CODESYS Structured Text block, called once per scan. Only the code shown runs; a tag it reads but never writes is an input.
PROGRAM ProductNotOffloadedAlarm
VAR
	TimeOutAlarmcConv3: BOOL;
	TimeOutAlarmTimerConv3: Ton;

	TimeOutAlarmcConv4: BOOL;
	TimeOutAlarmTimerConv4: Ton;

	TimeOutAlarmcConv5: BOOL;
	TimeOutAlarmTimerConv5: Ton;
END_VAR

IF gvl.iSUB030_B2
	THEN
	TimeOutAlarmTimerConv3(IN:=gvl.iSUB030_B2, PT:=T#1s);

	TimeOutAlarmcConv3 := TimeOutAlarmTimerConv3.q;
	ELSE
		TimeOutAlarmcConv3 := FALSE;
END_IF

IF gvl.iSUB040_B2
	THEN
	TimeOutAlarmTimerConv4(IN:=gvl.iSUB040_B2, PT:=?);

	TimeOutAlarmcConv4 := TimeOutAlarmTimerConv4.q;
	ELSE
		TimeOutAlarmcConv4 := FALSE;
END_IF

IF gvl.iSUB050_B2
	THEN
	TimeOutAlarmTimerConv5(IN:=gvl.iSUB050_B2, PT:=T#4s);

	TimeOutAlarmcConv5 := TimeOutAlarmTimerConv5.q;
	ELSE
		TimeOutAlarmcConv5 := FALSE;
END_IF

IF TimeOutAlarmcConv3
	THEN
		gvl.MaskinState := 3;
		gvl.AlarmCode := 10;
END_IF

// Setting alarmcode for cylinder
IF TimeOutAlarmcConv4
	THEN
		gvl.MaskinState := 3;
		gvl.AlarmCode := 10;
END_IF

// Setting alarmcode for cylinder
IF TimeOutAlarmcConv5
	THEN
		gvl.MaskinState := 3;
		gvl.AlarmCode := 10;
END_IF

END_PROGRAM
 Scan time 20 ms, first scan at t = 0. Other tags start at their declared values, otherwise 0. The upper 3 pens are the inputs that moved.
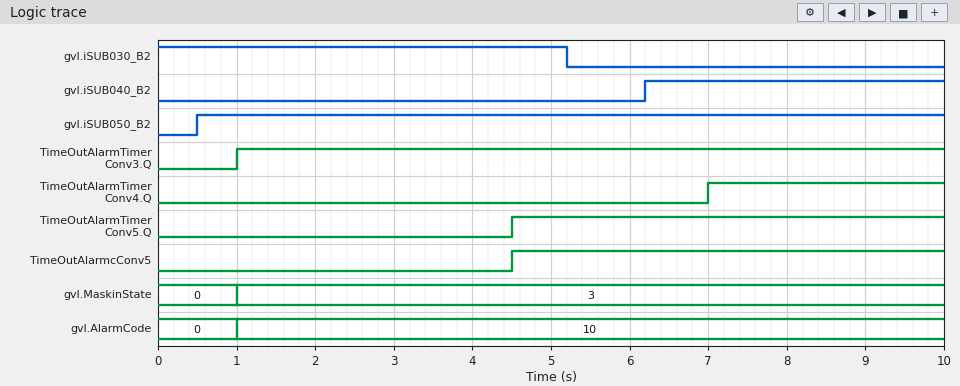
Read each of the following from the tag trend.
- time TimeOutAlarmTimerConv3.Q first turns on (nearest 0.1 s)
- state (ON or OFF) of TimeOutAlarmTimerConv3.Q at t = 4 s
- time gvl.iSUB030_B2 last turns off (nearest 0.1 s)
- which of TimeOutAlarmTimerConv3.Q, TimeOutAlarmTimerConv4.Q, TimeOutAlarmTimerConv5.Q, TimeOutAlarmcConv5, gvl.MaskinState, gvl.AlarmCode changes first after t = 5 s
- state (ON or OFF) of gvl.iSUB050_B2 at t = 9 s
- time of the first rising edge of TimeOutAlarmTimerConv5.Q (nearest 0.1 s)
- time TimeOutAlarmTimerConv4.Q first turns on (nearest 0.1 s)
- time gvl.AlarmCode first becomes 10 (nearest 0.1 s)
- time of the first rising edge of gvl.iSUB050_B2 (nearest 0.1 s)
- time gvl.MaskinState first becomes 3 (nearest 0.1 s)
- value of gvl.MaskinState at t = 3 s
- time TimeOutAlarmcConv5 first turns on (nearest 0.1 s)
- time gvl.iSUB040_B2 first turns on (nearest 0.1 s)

1.0 s
ON
5.2 s
TimeOutAlarmTimerConv4.Q
ON
4.5 s
7.0 s
1.0 s
0.5 s
1.0 s
3
4.5 s
6.2 s
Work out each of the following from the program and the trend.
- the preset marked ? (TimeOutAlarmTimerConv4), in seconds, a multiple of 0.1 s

0.8 s
